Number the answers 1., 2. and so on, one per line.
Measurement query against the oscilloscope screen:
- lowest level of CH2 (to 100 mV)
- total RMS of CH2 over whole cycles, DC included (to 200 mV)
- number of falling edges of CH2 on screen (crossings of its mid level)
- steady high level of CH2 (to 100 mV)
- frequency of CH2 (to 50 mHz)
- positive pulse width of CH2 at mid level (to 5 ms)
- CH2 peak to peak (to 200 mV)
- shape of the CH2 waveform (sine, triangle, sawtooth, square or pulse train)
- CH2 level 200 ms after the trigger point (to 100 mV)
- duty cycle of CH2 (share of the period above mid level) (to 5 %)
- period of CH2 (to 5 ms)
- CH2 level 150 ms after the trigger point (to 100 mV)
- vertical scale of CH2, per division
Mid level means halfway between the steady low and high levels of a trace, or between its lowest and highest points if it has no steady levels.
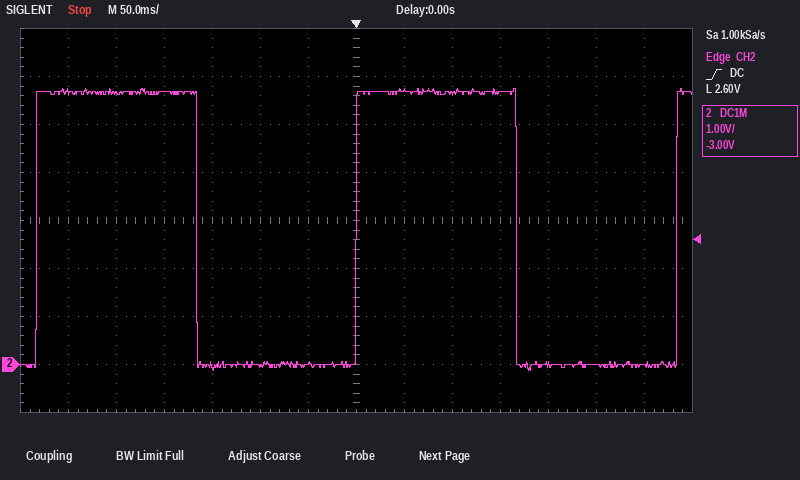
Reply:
1. -100 mV
2. 4.0 V
3. 2
4. 5.7 V
5. 3.00 Hz
6. 165 ms
7. 5.8 V
8. square
9. 0.0 V
10. 50 %
11. 335 ms
12. 5.7 V
13. 1 V
